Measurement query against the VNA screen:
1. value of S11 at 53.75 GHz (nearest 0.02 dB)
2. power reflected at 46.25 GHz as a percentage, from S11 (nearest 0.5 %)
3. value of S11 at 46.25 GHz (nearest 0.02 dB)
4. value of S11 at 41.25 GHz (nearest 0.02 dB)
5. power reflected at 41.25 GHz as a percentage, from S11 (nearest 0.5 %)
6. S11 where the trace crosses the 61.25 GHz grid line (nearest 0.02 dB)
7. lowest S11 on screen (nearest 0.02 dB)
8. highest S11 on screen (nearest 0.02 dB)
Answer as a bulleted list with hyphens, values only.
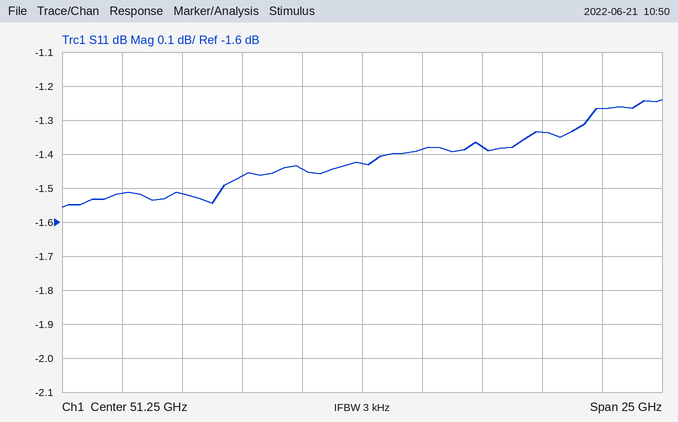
- -1.38 dB
- 71.5 %
- -1.46 dB
- -1.52 dB
- 70.5 %
- -1.26 dB
- -1.56 dB
- -1.24 dB
